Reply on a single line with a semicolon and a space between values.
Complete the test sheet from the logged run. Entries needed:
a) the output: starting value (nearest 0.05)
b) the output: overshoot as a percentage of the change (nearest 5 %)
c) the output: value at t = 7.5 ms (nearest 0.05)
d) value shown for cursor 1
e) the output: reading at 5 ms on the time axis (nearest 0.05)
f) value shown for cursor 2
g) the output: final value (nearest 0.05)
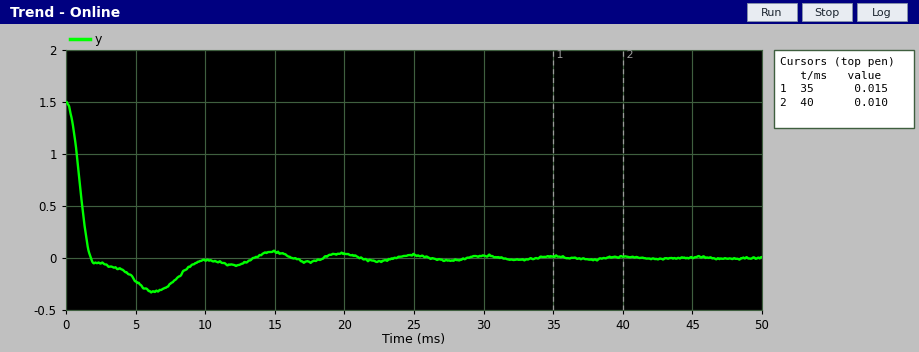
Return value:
1.50; 20 %; -0.25; 0.015; -0.20; 0.010; 0.00
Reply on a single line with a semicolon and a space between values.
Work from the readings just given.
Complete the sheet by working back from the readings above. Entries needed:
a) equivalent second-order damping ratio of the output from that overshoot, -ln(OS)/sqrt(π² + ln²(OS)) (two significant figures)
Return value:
0.46
